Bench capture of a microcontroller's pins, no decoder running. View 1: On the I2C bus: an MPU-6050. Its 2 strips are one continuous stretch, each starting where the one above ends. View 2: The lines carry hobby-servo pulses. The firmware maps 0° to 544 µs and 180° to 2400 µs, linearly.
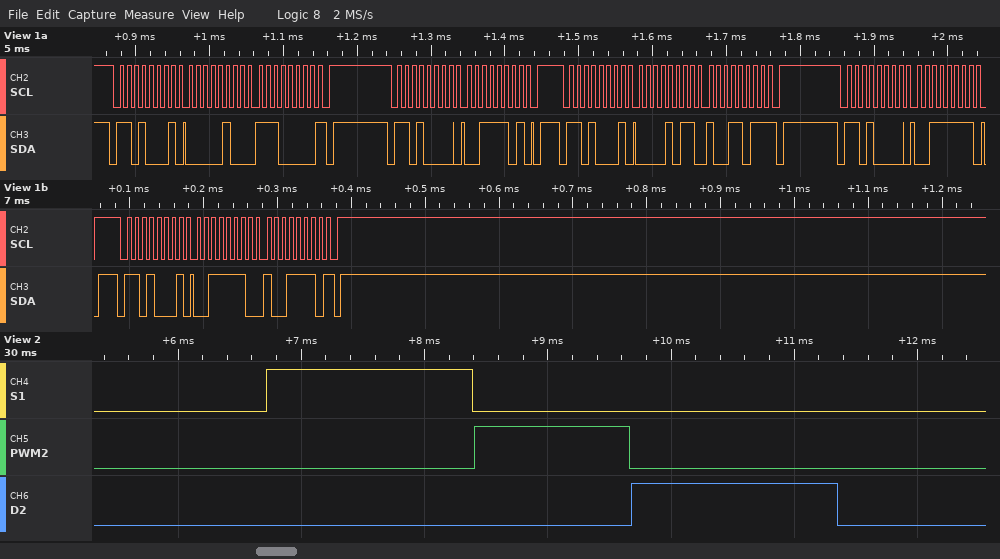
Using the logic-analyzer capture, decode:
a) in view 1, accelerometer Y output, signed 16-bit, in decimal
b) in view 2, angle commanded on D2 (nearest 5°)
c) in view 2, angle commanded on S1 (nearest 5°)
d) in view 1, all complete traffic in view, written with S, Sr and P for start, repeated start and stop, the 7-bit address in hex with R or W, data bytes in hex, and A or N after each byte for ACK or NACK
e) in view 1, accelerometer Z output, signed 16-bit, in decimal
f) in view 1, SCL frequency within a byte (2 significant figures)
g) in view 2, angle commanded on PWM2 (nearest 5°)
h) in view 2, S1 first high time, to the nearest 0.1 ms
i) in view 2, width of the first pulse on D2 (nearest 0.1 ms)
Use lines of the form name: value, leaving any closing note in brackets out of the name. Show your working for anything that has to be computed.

in view 1, accelerometer Y output, signed 16-bit, in decimal: 0x0B9B = 2971
in view 2, angle commanded on D2: 110°
in view 2, angle commanded on S1: 110°
in view 1, all complete traffic in view, written with S, Sr and P for start, repeated start and stop, the 7-bit address in hex with R or W, data bytes in hex, and A or N after each byte for ACK or NACK: S 68R A 04 A E0 N P S 68W A 3D A P S 68R A 0B A 9B N P S 68W A 3F A P S 68R A 3E A 9E N P
in view 1, accelerometer Z output, signed 16-bit, in decimal: 0x3E9E = 16030
in view 1, SCL frequency within a byte: 100 kHz
in view 2, angle commanded on PWM2: 70°
in view 2, S1 first high time, to the nearest 0.1 ms: 1.7 ms
in view 2, width of the first pulse on D2: 1.7 ms
